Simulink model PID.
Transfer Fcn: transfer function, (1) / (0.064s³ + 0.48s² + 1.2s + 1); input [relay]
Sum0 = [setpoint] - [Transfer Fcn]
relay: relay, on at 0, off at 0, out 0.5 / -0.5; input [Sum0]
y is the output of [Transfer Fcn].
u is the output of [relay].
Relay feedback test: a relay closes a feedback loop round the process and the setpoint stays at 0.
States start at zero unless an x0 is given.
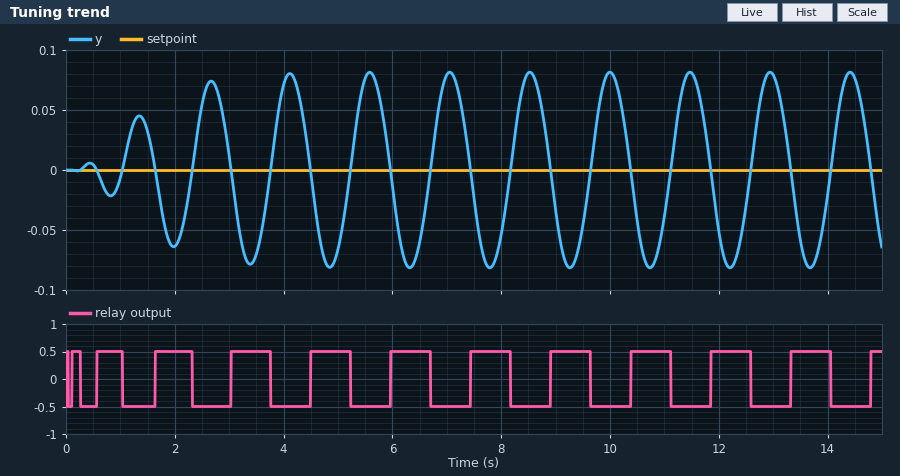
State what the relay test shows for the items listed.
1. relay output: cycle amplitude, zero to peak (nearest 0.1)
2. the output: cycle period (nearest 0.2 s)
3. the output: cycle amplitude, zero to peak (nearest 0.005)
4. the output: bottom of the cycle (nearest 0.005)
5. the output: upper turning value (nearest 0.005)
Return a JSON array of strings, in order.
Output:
["0.5", "1.4 s", "0.080", "-0.080", "0.080"]
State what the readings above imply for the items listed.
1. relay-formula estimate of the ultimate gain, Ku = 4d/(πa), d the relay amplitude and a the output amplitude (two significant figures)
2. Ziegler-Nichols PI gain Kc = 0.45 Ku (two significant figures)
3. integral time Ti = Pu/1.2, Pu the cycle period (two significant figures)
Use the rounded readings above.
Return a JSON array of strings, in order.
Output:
["8.0", "3.6", "1.2 s"]
